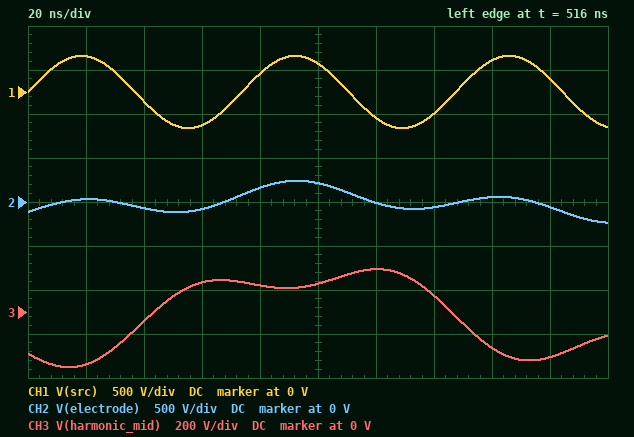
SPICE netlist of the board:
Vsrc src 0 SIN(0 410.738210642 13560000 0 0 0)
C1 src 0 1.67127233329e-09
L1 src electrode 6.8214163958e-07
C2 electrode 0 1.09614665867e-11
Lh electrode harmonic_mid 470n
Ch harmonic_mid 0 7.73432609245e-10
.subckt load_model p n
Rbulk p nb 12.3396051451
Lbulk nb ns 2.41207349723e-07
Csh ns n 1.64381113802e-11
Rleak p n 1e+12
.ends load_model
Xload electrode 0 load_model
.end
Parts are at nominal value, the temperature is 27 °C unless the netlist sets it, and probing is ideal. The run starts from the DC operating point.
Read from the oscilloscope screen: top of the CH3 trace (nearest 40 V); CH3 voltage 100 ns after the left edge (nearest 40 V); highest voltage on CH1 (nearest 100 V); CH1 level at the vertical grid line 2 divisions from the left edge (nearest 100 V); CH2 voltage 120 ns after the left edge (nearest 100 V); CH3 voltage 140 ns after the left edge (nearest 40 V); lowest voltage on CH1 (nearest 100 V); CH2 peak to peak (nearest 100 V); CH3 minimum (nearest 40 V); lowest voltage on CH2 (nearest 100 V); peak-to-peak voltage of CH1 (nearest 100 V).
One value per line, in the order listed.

200 V
120 V
400 V
-100 V
0 V
80 V
-400 V
500 V
-240 V
-200 V
800 V
